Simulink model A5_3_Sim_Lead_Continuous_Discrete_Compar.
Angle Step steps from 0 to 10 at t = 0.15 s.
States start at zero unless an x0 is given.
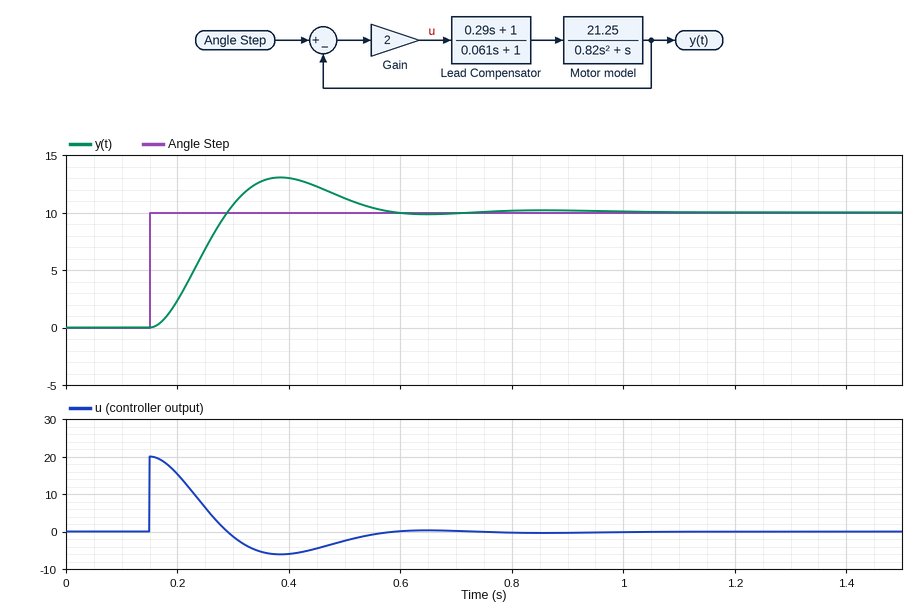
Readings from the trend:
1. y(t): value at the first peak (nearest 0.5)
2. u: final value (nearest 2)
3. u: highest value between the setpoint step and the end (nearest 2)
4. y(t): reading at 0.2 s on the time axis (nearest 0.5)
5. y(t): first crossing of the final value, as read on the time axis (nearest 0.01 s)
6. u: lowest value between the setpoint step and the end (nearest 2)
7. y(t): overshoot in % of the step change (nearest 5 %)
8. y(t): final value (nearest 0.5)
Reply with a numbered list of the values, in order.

1. 13.0
2. 0
3. 20
4. 2.5
5. 0.29 s
6. -6
7. 30 %
8. 10.0
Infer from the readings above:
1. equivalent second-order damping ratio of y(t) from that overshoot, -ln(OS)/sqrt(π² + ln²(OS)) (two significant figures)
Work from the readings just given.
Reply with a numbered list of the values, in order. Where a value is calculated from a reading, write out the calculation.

1. ln(0.3) = -1.204; 1.204 / sqrt(9.870 + 1.450) = 0.36
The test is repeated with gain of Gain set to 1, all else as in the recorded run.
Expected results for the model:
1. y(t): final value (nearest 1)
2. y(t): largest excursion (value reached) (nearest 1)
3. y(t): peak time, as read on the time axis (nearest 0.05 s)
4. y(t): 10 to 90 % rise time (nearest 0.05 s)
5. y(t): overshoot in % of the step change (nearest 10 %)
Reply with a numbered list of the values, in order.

1. 10
2. 12
3. 0.55 s
4. 0.15 s
5. 20 %
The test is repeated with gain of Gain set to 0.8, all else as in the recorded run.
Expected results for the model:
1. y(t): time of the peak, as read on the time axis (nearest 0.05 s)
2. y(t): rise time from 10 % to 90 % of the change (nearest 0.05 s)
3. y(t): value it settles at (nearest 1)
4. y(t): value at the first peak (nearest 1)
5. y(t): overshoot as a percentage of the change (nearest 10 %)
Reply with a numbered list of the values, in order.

1. 0.60 s
2. 0.20 s
3. 10
4. 12
5. 20 %
